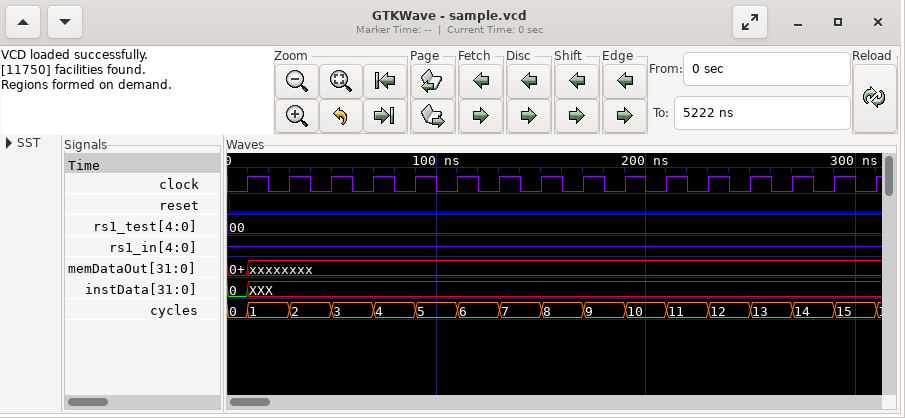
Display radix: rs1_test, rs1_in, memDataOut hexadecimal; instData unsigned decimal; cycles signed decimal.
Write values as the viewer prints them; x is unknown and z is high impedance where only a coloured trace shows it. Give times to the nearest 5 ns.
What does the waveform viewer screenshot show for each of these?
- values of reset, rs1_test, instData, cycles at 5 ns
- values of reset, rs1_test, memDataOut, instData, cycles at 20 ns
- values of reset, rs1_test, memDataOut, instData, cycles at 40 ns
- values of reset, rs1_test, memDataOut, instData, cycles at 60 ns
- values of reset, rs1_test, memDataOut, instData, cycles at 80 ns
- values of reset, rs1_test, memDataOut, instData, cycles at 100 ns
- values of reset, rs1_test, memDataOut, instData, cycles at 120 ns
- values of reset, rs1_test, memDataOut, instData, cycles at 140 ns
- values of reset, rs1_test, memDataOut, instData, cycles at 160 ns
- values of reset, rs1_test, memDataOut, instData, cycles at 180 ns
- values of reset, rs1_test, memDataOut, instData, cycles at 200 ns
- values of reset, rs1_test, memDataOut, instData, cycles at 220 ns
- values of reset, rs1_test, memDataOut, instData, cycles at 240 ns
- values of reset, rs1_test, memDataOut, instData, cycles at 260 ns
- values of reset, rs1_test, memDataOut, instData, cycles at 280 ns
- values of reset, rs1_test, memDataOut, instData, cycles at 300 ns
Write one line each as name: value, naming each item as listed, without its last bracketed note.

values of reset, rs1_test, instData, cycles at 5 ns: reset=0, rs1_test=00, instData=0, cycles=0
values of reset, rs1_test, memDataOut, instData, cycles at 20 ns: reset=0, rs1_test=00, memDataOut=xxxxxxxx, instData=XXX, cycles=1
values of reset, rs1_test, memDataOut, instData, cycles at 40 ns: reset=0, rs1_test=00, memDataOut=xxxxxxxx, instData=XXX, cycles=2
values of reset, rs1_test, memDataOut, instData, cycles at 60 ns: reset=0, rs1_test=00, memDataOut=xxxxxxxx, instData=XXX, cycles=3
values of reset, rs1_test, memDataOut, instData, cycles at 80 ns: reset=0, rs1_test=00, memDataOut=xxxxxxxx, instData=XXX, cycles=4
values of reset, rs1_test, memDataOut, instData, cycles at 100 ns: reset=0, rs1_test=00, memDataOut=xxxxxxxx, instData=XXX, cycles=5
values of reset, rs1_test, memDataOut, instData, cycles at 120 ns: reset=0, rs1_test=00, memDataOut=xxxxxxxx, instData=XXX, cycles=6
values of reset, rs1_test, memDataOut, instData, cycles at 140 ns: reset=0, rs1_test=00, memDataOut=xxxxxxxx, instData=XXX, cycles=7
values of reset, rs1_test, memDataOut, instData, cycles at 160 ns: reset=0, rs1_test=00, memDataOut=xxxxxxxx, instData=XXX, cycles=8
values of reset, rs1_test, memDataOut, instData, cycles at 180 ns: reset=0, rs1_test=00, memDataOut=xxxxxxxx, instData=XXX, cycles=9
values of reset, rs1_test, memDataOut, instData, cycles at 200 ns: reset=0, rs1_test=00, memDataOut=xxxxxxxx, instData=XXX, cycles=10
values of reset, rs1_test, memDataOut, instData, cycles at 220 ns: reset=0, rs1_test=00, memDataOut=xxxxxxxx, instData=XXX, cycles=11
values of reset, rs1_test, memDataOut, instData, cycles at 240 ns: reset=0, rs1_test=00, memDataOut=xxxxxxxx, instData=XXX, cycles=12
values of reset, rs1_test, memDataOut, instData, cycles at 260 ns: reset=0, rs1_test=00, memDataOut=xxxxxxxx, instData=XXX, cycles=13
values of reset, rs1_test, memDataOut, instData, cycles at 280 ns: reset=0, rs1_test=00, memDataOut=xxxxxxxx, instData=XXX, cycles=14
values of reset, rs1_test, memDataOut, instData, cycles at 300 ns: reset=0, rs1_test=00, memDataOut=xxxxxxxx, instData=XXX, cycles=15
